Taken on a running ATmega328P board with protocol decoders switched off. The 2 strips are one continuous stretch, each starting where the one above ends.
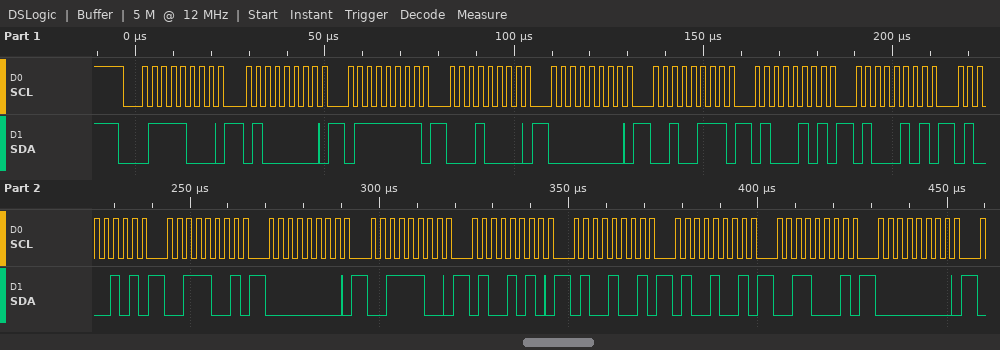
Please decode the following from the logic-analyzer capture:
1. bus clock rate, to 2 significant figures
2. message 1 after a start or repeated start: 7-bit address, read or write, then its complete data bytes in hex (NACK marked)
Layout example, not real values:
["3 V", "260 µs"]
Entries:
["400 kHz", "0x3C write: 40 7F 10 00 27 45 45 45 39 00 3C 4A 49 49 31 00"]
